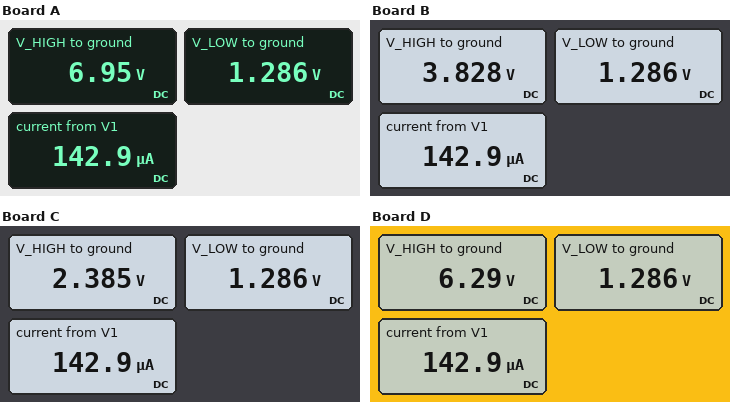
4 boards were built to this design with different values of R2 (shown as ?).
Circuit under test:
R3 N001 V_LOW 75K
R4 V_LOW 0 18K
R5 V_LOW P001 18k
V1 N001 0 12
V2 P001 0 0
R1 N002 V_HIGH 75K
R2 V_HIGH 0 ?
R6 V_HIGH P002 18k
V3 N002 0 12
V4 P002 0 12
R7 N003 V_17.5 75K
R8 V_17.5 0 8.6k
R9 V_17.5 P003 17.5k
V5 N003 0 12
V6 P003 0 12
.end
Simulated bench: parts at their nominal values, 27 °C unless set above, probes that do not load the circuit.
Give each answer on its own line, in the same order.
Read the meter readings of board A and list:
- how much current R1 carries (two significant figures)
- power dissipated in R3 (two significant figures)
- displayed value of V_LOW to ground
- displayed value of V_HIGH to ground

67 µA
1.5 mW
1.286 V
6.95 V
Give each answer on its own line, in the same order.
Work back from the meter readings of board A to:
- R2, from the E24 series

20 kΩ
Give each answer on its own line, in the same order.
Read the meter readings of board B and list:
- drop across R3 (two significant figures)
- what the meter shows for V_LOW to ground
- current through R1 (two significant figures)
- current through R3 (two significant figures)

11 V
1.286 V
110 µA
140 µA
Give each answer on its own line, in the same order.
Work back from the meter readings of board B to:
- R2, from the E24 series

6.8 kΩ
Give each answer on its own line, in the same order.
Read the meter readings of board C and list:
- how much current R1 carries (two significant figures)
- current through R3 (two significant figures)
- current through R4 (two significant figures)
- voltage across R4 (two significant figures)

130 µA
140 µA
71 µA
1.3 V
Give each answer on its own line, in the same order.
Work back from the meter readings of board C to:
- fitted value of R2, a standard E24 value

3.6 kΩ
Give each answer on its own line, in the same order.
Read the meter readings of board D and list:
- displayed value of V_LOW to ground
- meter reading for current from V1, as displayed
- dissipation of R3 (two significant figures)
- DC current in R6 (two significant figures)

1.286 V
142.9 µA
1.5 mW
320 µA
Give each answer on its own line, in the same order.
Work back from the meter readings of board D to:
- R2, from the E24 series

16 kΩ
